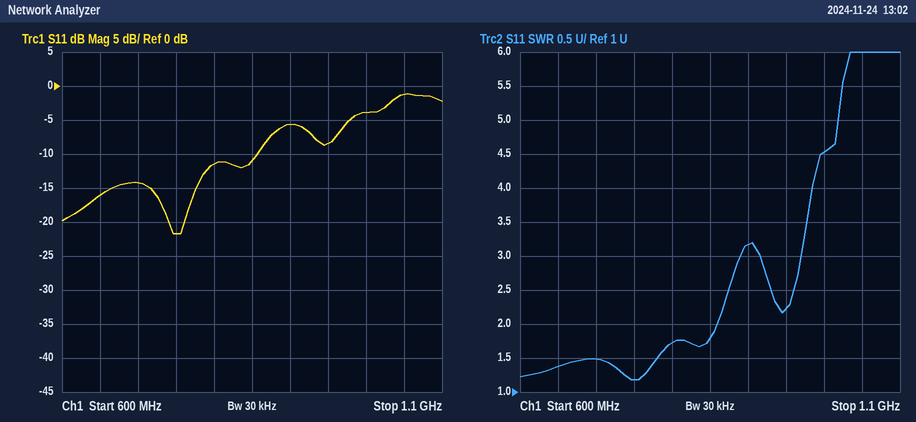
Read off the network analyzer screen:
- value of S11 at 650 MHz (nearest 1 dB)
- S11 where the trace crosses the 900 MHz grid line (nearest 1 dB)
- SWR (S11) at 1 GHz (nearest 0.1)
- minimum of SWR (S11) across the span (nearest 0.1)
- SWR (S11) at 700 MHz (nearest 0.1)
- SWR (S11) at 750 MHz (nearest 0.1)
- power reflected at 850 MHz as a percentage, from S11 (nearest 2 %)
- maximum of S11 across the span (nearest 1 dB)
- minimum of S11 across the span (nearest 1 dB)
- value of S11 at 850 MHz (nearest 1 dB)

-16 dB
-6 dB
4.5
1.2
1.5
1.2
8 %
-1 dB
-22 dB
-11 dB
